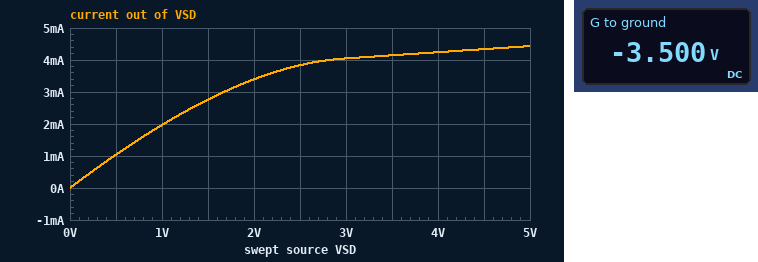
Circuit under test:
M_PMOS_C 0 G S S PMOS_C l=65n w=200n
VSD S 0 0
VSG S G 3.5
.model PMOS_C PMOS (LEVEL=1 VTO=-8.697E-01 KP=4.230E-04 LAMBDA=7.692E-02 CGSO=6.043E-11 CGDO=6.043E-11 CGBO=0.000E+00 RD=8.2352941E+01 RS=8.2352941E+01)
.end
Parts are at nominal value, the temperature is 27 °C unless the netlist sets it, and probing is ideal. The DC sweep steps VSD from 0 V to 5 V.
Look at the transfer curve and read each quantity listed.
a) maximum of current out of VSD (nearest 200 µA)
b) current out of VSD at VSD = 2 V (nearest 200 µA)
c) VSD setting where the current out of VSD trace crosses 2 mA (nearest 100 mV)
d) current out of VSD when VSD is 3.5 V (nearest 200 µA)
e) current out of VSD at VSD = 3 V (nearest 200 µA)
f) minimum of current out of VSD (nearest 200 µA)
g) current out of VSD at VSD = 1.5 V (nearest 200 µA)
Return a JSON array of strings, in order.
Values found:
["4.4 mA", "3.4 mA", "1.0 V", "4.2 mA", "4.0 mA", "0 A", "2.8 mA"]
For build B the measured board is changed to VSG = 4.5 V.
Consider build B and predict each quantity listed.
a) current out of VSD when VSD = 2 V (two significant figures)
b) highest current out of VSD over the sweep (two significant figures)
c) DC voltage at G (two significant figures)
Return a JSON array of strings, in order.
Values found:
["4.6 mA", "7.6 mA", "-4.5 V"]
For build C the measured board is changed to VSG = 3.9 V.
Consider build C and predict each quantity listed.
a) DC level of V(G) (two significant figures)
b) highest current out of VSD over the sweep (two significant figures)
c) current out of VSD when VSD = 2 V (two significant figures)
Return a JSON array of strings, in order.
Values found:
["-3.9 V", "5.6 mA", "3.9 mA"]
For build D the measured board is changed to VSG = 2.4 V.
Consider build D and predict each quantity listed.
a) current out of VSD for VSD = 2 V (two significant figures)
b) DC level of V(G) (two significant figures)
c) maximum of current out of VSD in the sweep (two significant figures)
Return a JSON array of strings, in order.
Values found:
["1.5 mA", "-2.4 V", "1.7 mA"]
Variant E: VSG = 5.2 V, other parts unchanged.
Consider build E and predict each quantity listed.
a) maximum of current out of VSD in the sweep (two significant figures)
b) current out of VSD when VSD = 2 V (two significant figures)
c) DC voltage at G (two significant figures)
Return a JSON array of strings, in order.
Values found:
["10 mA", "5.3 mA", "-5.2 V"]
